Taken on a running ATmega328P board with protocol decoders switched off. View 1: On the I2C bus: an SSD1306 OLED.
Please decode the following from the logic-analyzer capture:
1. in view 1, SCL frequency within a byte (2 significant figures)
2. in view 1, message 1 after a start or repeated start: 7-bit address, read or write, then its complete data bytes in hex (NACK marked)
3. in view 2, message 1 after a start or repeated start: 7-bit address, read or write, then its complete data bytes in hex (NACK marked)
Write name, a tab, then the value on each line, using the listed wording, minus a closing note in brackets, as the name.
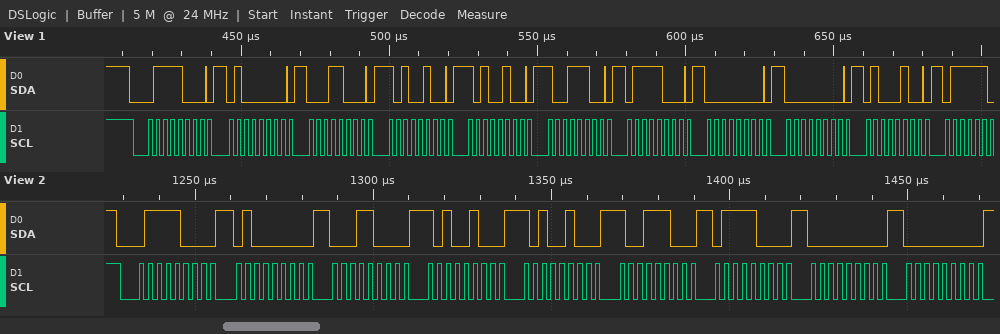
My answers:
in view 1, SCL frequency within a byte	400 kHz
in view 1, message 1 after a start or repeated start: 7-bit address, read or write, then its complete data bytes in hex	0x3C write: 40 18 A4 A4 9C 78 00 00 44
in view 2, message 1 after a start or repeated start: 7-bit address, read or write, then its complete data bytes in hex	0x3C write: 40 18 A4 A4 9C 78 00 00
